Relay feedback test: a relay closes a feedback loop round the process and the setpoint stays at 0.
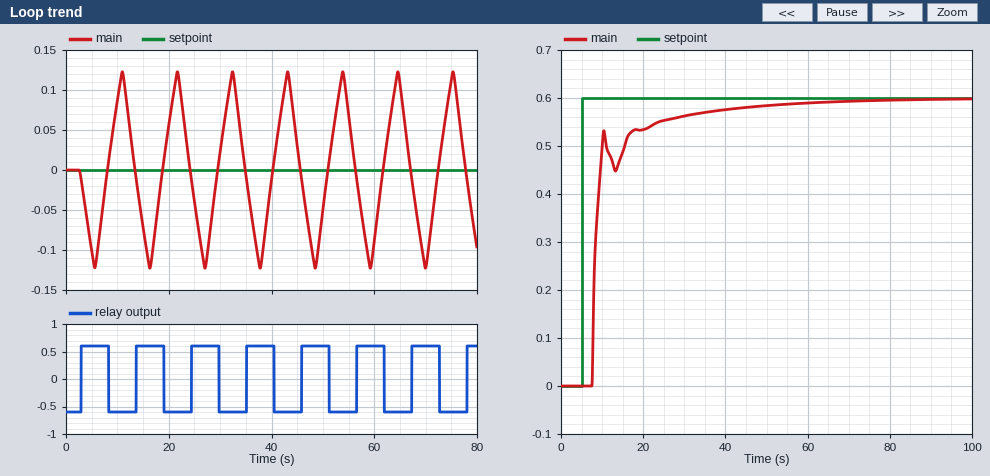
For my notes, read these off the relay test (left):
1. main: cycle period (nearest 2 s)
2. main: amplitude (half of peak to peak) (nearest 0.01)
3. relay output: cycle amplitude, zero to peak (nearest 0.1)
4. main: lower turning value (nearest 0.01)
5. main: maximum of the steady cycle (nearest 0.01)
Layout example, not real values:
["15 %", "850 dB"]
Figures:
["10 s", "0.12", "0.6", "-0.12", "0.12"]
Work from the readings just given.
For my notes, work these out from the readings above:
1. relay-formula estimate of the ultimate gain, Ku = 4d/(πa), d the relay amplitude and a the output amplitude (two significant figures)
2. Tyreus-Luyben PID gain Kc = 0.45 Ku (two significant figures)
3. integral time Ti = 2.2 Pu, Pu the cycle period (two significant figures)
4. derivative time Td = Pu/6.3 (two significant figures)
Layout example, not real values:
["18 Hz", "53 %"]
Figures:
["6.4", "2.9", "22 s", "1.6 s"]
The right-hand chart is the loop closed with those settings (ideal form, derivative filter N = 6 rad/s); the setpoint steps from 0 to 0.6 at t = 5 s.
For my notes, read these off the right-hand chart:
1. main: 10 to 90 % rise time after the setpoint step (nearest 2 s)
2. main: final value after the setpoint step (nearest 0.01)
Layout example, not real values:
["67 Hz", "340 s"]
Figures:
["14 s", "0.60"]
